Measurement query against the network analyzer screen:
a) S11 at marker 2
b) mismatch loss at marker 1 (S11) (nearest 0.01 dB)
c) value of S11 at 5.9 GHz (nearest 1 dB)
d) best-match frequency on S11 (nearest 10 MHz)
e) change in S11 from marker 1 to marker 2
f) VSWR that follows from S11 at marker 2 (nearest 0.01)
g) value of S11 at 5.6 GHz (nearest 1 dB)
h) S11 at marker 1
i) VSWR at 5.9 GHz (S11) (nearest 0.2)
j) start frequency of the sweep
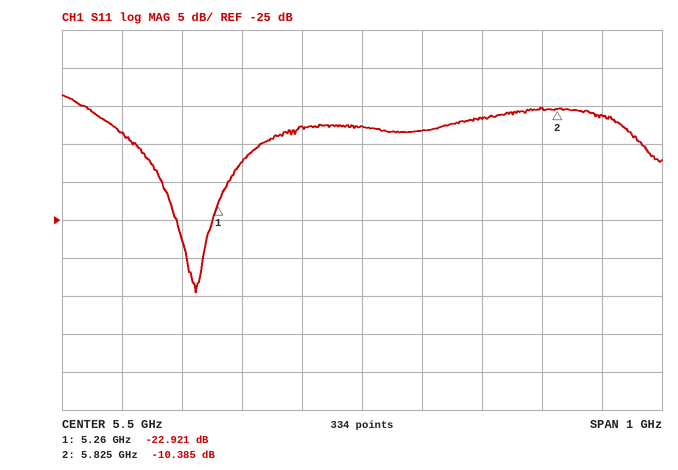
-10.385 dB
0.02 dB
-11 dB
5.22 GHz
12.536 dB
1.87
-13 dB
-22.921 dB
1.8
5 GHz
